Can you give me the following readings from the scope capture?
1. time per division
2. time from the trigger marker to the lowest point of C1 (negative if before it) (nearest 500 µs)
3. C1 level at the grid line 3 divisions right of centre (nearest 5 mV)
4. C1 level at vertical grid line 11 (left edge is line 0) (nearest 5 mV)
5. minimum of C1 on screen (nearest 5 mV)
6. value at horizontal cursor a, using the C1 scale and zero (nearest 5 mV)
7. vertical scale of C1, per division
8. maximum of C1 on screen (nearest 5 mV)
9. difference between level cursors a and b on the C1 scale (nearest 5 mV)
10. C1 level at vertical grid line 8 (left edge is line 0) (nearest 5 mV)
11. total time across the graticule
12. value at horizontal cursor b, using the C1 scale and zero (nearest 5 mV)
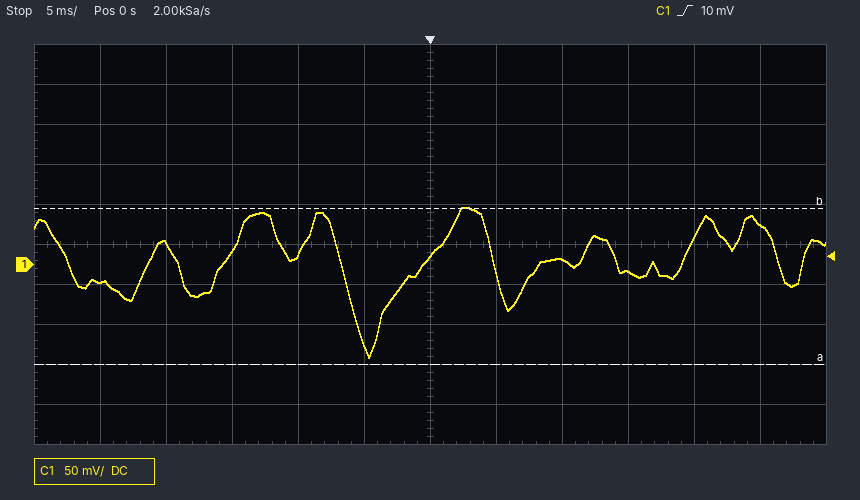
5 ms
-4.5 ms
-10 mV
50 mV
-115 mV
-125 mV
50 mV
70 mV
195 mV
5 mV
60 ms
70 mV
